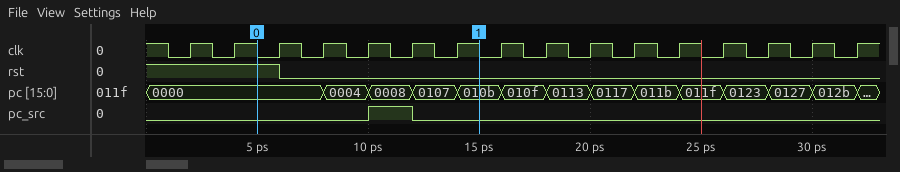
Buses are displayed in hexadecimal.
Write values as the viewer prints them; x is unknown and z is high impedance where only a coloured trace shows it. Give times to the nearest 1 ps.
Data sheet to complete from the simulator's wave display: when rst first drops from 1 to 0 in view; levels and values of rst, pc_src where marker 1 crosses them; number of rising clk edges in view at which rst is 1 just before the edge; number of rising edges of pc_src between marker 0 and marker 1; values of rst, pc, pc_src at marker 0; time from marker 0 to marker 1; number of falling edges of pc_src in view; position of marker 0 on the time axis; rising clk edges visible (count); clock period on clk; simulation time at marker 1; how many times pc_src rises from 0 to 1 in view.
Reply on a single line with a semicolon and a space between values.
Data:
6 ps; rst=0, pc_src=0; 3; 1; rst=1, pc=0000, pc_src=0; 10 ps; 1; 5 ps; 16; 2 ps; 15 ps; 1
